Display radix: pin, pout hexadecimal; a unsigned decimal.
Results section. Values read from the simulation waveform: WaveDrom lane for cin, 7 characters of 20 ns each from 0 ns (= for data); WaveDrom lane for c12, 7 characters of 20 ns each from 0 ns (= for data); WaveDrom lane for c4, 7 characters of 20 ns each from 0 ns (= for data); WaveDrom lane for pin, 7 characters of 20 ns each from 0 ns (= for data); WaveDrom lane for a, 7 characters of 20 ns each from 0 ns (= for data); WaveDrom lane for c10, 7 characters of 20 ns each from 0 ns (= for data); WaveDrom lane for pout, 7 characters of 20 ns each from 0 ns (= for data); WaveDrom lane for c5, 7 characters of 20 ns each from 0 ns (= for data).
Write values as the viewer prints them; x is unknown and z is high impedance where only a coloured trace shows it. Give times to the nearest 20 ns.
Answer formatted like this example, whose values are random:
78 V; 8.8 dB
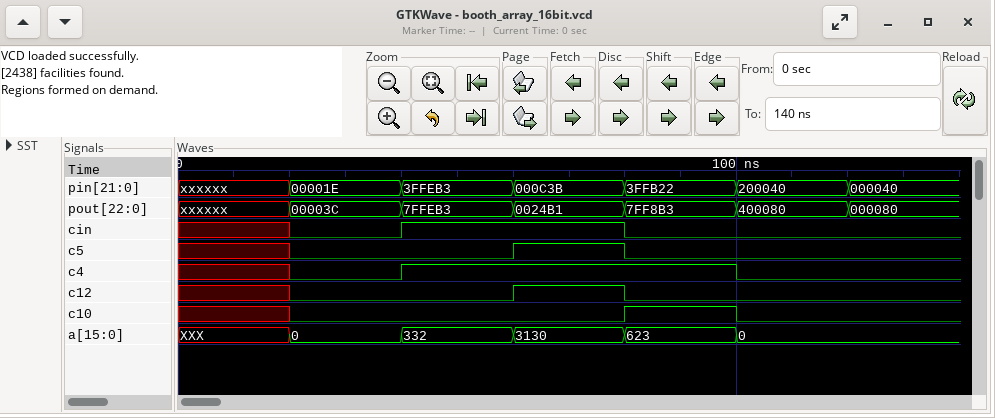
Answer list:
{name: 'cin', wave: 'x01.0..'}; {name: 'c12', wave: 'x0.10..'}; {name: 'c4', wave: 'x01..0.'}; {name: 'pin', wave: 'x======', data: '00001E 3FFEB3 000C3B 3FFB22 200040 000040'}; {name: 'a', wave: 'x=====.', data: '0 332 3130 623 0'}; {name: 'c10', wave: 'x0..10.'}; {name: 'pout', wave: 'x======', data: '00003C 7FFEB3 0024B1 7FF8B3 400080 000080'}; {name: 'c5', wave: 'x0.10..'}
